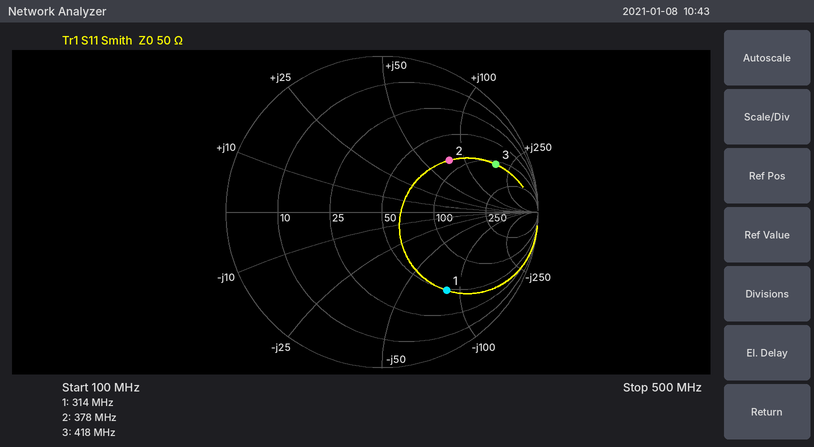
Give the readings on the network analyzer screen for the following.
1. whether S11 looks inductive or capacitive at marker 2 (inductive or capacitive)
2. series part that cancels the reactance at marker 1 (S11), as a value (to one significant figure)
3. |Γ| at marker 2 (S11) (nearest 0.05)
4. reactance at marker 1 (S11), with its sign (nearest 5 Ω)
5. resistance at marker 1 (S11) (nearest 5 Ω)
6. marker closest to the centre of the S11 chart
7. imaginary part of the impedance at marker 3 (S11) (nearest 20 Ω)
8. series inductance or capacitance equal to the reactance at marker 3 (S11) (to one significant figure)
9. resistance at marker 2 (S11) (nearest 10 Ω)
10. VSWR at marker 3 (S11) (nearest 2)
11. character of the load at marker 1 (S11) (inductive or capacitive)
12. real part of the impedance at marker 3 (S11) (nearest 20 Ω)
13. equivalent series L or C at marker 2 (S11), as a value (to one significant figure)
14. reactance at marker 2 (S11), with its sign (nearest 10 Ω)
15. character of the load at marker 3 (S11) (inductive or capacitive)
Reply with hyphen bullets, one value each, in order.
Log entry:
- inductive
- 40 nH
- 0.55
- -85 Ω
- 50 Ω
- marker 2
- +180 Ω
- 70 nH
- 80 Ω
- 8
- capacitive
- 120 Ω
- 30 nH
- +80 Ω
- inductive
